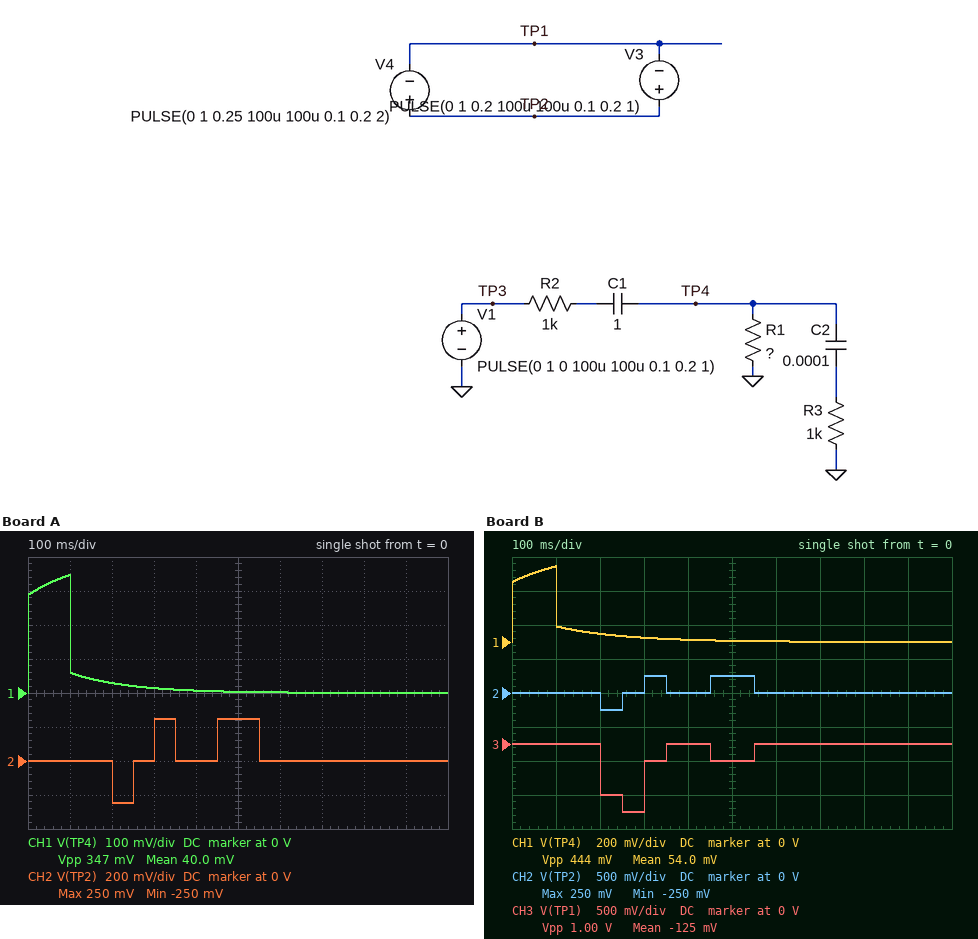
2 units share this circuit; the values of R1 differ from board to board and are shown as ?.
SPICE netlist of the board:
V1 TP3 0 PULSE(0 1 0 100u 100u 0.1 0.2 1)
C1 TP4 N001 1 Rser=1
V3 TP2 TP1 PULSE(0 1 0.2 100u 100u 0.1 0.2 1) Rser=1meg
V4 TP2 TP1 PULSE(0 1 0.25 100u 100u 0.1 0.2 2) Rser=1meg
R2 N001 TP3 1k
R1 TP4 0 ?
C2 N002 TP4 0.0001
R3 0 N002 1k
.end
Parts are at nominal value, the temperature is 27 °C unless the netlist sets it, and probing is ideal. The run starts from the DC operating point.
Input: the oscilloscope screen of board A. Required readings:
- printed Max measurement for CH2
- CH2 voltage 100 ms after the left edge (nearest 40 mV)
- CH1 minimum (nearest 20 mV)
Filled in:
250 mV
0 V
0 V
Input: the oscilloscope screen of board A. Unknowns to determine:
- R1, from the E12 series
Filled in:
680 Ω
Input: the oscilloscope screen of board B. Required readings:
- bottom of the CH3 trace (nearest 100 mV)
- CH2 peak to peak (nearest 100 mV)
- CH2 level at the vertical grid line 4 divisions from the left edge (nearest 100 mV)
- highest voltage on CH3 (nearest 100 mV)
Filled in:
-1.0 V
500 mV
0 V
0 V
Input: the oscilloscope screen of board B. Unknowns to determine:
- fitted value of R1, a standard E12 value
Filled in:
1.2 kΩ
